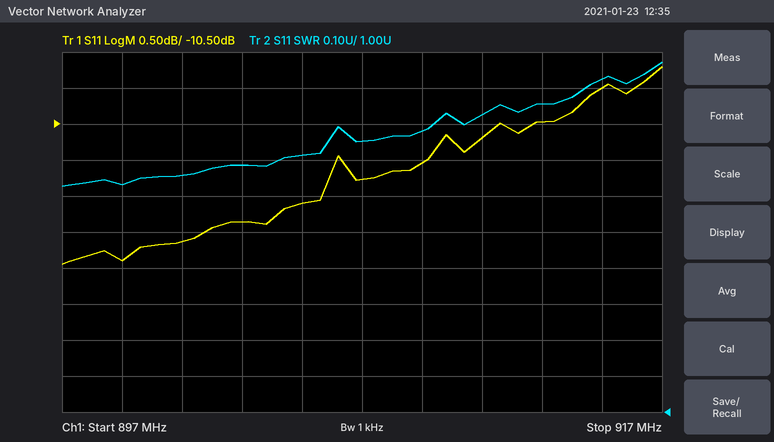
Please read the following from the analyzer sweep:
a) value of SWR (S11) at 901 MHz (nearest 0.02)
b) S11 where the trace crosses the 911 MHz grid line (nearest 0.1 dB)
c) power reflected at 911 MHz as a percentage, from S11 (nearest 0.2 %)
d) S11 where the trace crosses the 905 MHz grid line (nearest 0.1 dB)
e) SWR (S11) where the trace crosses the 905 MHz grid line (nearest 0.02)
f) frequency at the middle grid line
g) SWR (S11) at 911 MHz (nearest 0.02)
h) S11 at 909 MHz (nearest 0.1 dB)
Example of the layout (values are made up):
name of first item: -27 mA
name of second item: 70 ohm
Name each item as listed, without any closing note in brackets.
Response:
value of SWR (S11) at 901 MHz: 1.66
S11 where the trace crosses the 911 MHz grid line: -10.7 dB
power reflected at 911 MHz as a percentage, from S11: 8.6 %
S11 where the trace crosses the 905 MHz grid line: -11.6 dB
SWR (S11) where the trace crosses the 905 MHz grid line: 1.72
frequency at the middle grid line: 907 MHz
SWR (S11) at 911 MHz: 1.82
S11 at 909 MHz: -11.0 dB
